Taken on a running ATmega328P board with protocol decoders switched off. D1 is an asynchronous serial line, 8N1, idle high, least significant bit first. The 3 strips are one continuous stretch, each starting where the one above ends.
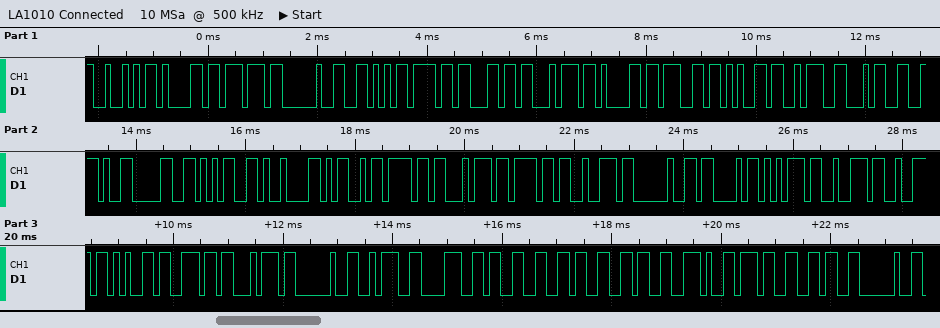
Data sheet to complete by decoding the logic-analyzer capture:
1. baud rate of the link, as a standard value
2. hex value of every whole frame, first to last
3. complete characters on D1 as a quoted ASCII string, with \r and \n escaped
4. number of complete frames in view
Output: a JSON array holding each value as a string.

["9600 baud", "0x52 0x61 0x77 0x20 0x56 0x6F 0x6C 0x74 0x61 0x67 0x65 0x3A 0x34 0x2E 0x30 0x35 0x09 0x4D 0x6F 0x74 0x6F 0x72 0x20 0x43 0x75 0x72 0x72 0x65 0x6E 0x74 0x20 0x3A 0x38 0x33 0x36 0x36 0x2E 0x37 0x36 0x20", "\"Raw Voltage:4.05\\tMotor Current :8366.76 \"", "40"]
